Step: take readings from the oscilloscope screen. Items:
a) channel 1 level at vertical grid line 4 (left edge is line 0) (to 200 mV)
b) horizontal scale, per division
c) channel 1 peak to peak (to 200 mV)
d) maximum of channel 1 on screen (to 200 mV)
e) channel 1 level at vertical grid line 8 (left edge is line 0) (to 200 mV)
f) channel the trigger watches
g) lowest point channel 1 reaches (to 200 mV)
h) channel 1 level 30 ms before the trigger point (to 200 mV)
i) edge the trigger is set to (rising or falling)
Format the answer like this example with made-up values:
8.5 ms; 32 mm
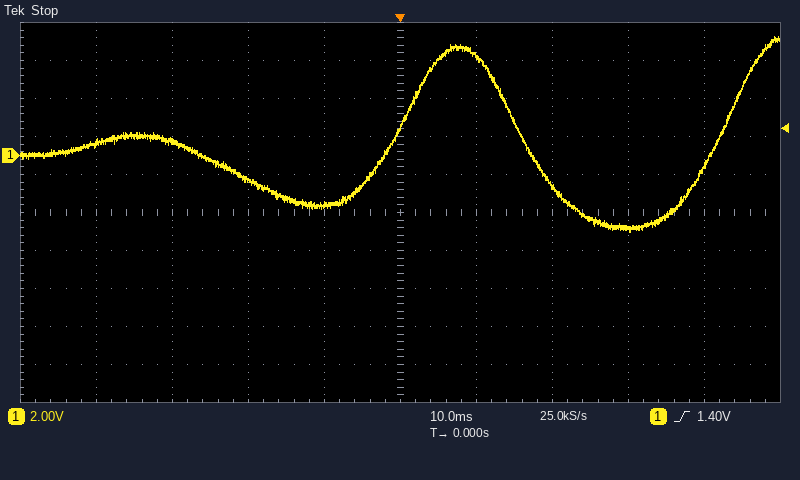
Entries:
-2.6 V; 10 ms; 10.2 V; 6.2 V; -3.8 V; channel 1; -4.0 V; 800 mV; rising
